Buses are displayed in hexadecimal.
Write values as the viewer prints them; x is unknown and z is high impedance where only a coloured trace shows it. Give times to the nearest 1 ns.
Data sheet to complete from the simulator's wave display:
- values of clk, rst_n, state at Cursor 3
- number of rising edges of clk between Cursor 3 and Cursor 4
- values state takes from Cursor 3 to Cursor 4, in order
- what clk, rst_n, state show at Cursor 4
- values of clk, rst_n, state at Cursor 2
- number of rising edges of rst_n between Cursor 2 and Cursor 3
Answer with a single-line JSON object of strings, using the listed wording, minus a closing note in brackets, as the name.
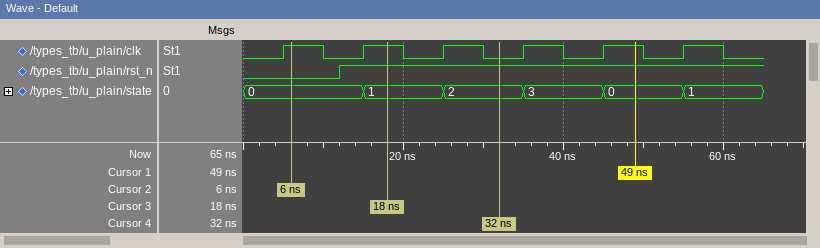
{"values of clk, rst_n, state at Cursor 3": "clk=1, rst_n=1, state=1", "number of rising edges of clk between Cursor 3 and Cursor 4": "1", "values state takes from Cursor 3 to Cursor 4, in order": "1, 2", "what clk, rst_n, state show at Cursor 4": "clk=0, rst_n=1, state=2", "values of clk, rst_n, state at Cursor 2": "clk=1, rst_n=0, state=0", "number of rising edges of rst_n between Cursor 2 and Cursor 3": "1"}
